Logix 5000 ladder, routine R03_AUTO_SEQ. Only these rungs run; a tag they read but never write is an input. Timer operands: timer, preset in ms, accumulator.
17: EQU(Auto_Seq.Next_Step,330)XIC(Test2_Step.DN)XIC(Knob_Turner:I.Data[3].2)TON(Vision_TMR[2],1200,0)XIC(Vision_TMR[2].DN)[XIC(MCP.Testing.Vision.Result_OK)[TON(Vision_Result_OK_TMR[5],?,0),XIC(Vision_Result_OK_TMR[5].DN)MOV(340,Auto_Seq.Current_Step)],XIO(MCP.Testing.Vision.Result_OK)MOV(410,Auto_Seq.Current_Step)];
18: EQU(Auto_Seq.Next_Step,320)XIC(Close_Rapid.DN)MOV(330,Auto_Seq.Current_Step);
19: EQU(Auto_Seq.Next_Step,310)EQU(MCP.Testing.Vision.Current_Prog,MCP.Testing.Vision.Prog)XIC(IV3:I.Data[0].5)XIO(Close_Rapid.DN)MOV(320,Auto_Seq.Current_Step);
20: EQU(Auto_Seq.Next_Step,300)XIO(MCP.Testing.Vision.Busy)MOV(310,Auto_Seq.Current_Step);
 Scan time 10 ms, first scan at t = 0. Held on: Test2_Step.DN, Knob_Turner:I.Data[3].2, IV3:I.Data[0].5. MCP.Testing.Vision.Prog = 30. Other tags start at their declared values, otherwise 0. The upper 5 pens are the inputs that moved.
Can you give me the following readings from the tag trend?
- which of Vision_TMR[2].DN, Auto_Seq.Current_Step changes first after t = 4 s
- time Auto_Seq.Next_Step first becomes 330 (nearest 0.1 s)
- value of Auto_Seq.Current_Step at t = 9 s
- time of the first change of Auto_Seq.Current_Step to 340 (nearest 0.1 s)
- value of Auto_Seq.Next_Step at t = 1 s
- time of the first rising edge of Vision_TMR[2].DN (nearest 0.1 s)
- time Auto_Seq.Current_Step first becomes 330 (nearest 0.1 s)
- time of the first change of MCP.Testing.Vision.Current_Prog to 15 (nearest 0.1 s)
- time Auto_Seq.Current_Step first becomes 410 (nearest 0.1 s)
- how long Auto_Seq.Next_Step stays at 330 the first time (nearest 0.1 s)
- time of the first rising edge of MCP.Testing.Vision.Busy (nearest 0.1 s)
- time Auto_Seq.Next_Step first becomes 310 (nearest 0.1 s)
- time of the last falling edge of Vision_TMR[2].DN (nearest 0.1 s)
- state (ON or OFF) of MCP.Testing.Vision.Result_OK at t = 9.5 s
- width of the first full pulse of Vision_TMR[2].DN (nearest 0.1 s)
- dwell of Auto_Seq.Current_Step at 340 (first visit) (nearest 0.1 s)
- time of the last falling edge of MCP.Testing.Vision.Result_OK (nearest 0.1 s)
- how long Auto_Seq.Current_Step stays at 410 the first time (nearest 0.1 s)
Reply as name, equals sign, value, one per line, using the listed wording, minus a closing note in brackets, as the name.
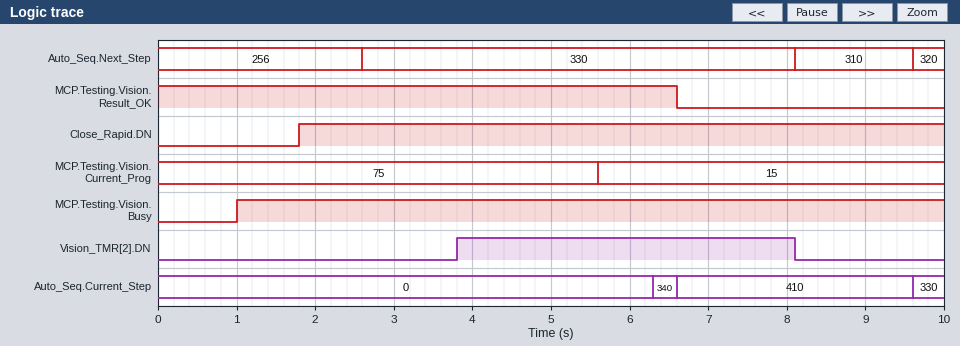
which of Vision_TMR[2].DN, Auto_Seq.Current_Step changes first after t = 4 s = Auto_Seq.Current_Step
time Auto_Seq.Next_Step first becomes 330 = 2.6 s
value of Auto_Seq.Current_Step at t = 9 s = 410
time of the first change of Auto_Seq.Current_Step to 340 = 6.3 s
value of Auto_Seq.Next_Step at t = 1 s = 256
time of the first rising edge of Vision_TMR[2].DN = 3.8 s
time Auto_Seq.Current_Step first becomes 330 = 9.6 s
time of the first change of MCP.Testing.Vision.Current_Prog to 15 = 5.6 s
time Auto_Seq.Current_Step first becomes 410 = 6.6 s
how long Auto_Seq.Next_Step stays at 330 the first time = 5.5 s
time of the first rising edge of MCP.Testing.Vision.Busy = 1.0 s
time Auto_Seq.Next_Step first becomes 310 = 8.1 s
time of the last falling edge of Vision_TMR[2].DN = 8.1 s
state (ON or OFF) of MCP.Testing.Vision.Result_OK at t = 9.5 s = OFF
width of the first full pulse of Vision_TMR[2].DN = 4.3 s
dwell of Auto_Seq.Current_Step at 340 (first visit) = 0.3 s
time of the last falling edge of MCP.Testing.Vision.Result_OK = 6.6 s
how long Auto_Seq.Current_Step stays at 410 the first time = 3.0 s
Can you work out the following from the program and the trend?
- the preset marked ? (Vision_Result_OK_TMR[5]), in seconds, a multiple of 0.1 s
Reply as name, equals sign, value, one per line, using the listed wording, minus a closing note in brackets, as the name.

the preset marked ? (Vision_Result_OK_TMR[5]), in seconds, a multiple of 0.1 s = 2.5 s
